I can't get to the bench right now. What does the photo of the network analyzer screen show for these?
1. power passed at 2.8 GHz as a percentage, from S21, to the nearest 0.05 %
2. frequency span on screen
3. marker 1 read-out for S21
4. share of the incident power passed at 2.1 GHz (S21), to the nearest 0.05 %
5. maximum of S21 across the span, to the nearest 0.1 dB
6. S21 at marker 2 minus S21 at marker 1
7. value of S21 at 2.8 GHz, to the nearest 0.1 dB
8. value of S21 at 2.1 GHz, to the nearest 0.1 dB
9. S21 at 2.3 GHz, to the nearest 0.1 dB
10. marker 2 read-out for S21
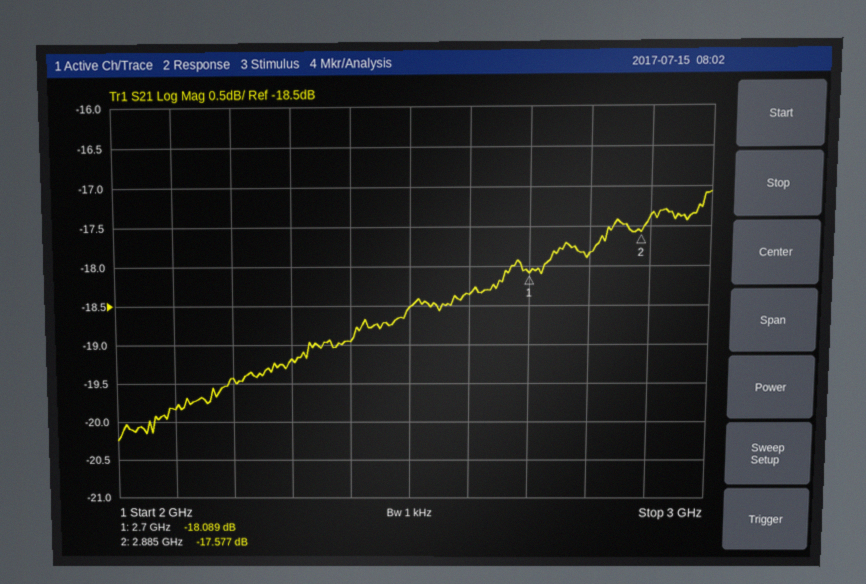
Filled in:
1.65 %
1 GHz
-18.089 dB
1.05 %
-17.1 dB
0.512 dB
-17.8 dB
-19.8 dB
-19.2 dB
-17.577 dB
